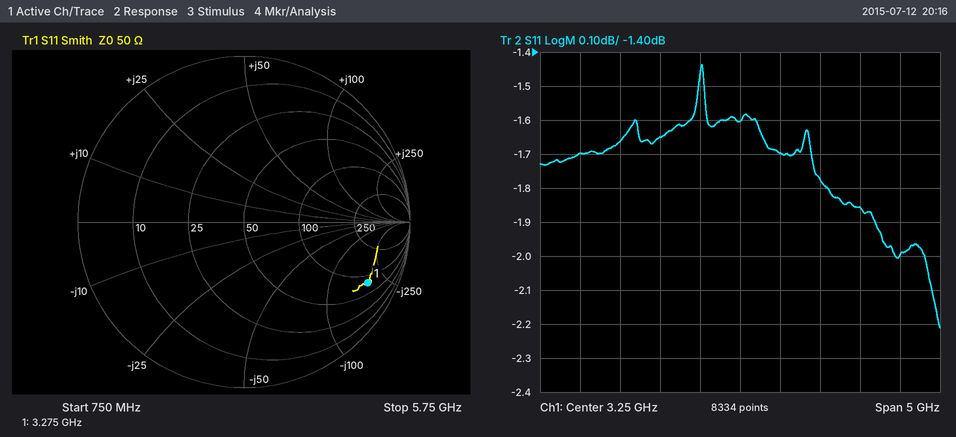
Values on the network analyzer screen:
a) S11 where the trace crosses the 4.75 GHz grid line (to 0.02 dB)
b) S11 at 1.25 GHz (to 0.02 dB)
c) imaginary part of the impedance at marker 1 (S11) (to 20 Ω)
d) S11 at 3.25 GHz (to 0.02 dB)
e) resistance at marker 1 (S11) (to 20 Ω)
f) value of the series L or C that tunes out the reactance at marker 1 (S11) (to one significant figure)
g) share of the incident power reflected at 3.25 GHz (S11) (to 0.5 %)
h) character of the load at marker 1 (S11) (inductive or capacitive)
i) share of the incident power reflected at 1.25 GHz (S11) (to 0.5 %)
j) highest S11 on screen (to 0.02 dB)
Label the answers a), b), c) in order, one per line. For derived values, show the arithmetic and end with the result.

a) -1.86 dB
b) -1.70 dB
c) -180 Ω
d) -1.60 dB
e) 80 Ω
f) L = 180 Ω/(2π × 3.275 GHz) ≈ 9 nH
g) 10^(-1.6/10) ≈ 69.2 %, so 69.0 % to the nearest 0.5 %
h) capacitive
i) 10^(-1.7/10) ≈ 67.6 %, so 67.5 % to the nearest 0.5 %
j) -1.44 dB
